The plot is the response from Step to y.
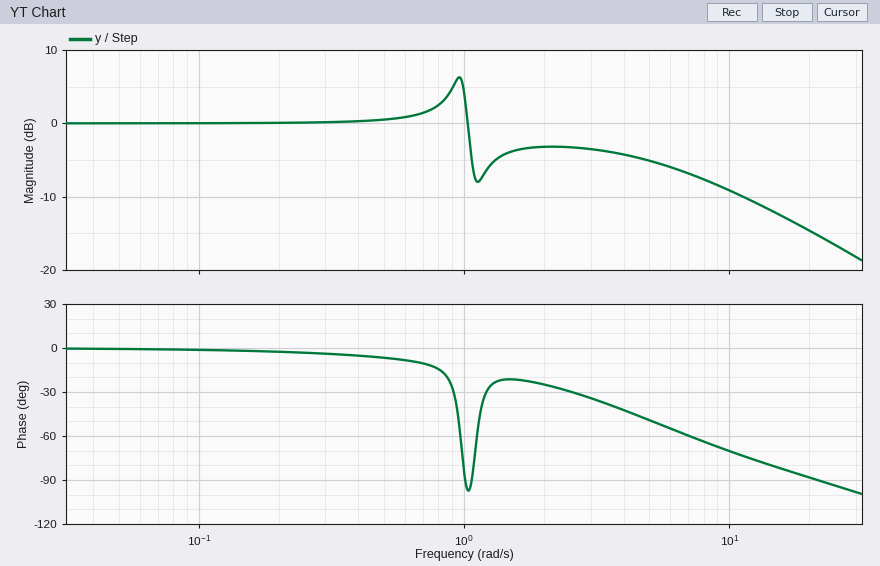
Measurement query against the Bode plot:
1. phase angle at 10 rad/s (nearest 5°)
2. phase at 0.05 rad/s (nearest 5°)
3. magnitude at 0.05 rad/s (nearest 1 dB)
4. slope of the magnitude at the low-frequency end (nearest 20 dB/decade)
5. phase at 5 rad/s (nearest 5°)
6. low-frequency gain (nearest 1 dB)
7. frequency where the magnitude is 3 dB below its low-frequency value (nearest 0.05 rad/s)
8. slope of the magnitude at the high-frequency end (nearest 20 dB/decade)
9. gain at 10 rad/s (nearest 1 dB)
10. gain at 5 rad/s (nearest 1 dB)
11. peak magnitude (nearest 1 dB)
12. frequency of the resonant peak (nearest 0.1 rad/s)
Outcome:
-70°
0°
0 dB
0 dB/decade
-50°
0 dB
1.05 rad/s
-20 dB/decade
-9 dB
-5 dB
6 dB
1.0 rad/s
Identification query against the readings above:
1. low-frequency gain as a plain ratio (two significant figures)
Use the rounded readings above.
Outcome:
1.0
